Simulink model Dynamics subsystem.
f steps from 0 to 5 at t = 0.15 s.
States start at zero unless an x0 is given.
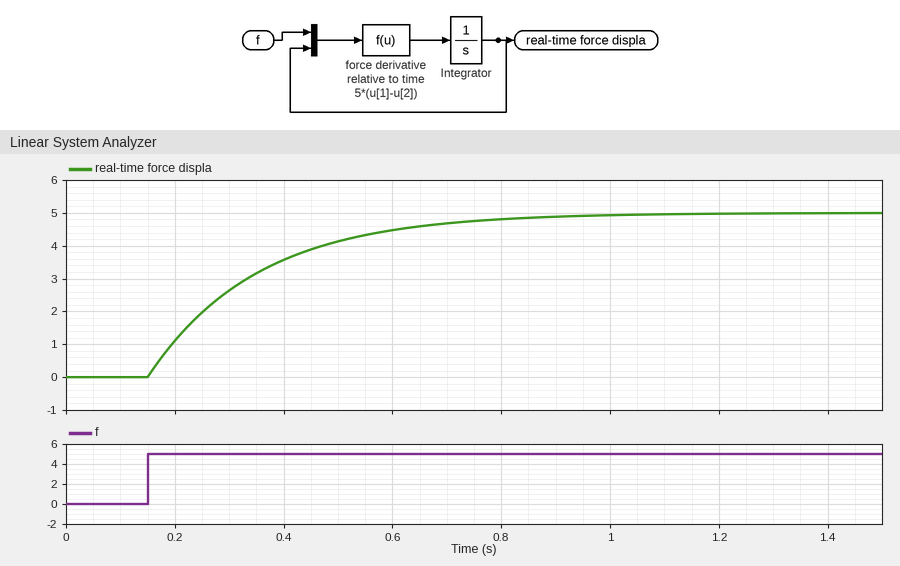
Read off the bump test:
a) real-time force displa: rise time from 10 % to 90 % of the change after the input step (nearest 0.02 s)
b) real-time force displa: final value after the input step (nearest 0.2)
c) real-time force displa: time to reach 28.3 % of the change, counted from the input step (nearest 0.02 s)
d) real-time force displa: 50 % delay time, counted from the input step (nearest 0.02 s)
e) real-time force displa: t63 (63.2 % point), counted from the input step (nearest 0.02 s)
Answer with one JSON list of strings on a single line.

["0.44 s", "5.0", "0.06 s", "0.14 s", "0.20 s"]
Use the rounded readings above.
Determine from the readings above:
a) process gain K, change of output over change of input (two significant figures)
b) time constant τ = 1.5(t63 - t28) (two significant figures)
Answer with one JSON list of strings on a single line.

["1.0", "0.21 s"]
